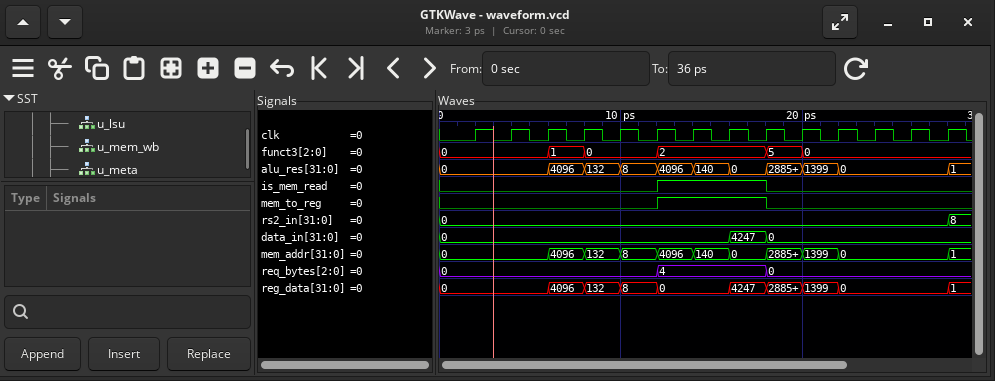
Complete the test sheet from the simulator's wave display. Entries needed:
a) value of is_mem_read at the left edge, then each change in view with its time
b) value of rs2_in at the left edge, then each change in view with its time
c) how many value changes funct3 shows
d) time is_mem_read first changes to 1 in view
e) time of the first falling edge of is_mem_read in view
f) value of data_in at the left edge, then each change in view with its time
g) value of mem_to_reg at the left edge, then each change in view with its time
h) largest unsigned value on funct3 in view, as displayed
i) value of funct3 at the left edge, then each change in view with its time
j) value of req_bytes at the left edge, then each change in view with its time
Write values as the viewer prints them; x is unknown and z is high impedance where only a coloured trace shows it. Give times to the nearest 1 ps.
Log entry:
0, 1 at 12 ps, 0 at 18 ps
0, 8 at 28 ps
5
12 ps
18 ps
0, 4247 at 16 ps, 0 at 18 ps
0, 1 at 12 ps, 0 at 18 ps
5
0, 1 at 6 ps, 0 at 8 ps, 2 at 12 ps, 5 at 18 ps, 0 at 20 ps
0, 4 at 12 ps, 0 at 18 ps
